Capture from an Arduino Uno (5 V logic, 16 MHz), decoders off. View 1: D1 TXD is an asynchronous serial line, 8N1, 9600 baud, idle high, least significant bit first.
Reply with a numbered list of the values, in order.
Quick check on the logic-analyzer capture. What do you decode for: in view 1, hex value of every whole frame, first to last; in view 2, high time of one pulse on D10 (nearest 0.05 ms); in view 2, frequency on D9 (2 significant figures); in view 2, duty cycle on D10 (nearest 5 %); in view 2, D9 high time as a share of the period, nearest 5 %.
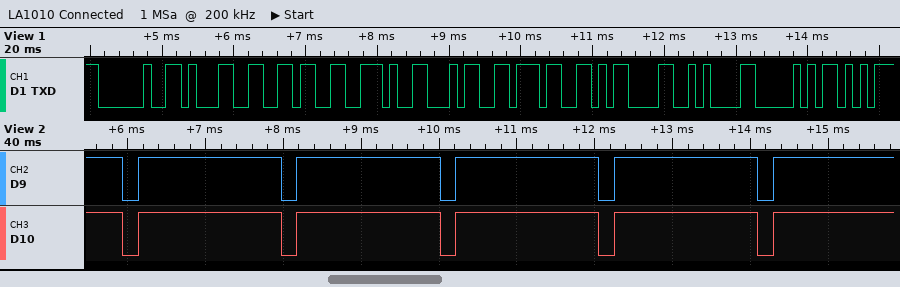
1. 0x20 0x31 0x36 0x2E 0x34 0x37 0x0D 0x0A 0x50
2. 1.85 ms
3. 490 Hz
4. 90 %
5. 90 %
